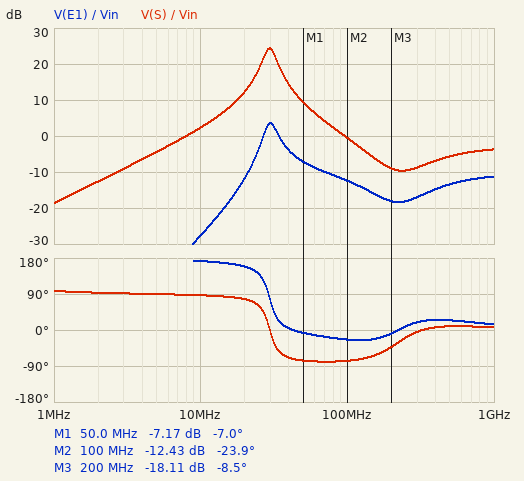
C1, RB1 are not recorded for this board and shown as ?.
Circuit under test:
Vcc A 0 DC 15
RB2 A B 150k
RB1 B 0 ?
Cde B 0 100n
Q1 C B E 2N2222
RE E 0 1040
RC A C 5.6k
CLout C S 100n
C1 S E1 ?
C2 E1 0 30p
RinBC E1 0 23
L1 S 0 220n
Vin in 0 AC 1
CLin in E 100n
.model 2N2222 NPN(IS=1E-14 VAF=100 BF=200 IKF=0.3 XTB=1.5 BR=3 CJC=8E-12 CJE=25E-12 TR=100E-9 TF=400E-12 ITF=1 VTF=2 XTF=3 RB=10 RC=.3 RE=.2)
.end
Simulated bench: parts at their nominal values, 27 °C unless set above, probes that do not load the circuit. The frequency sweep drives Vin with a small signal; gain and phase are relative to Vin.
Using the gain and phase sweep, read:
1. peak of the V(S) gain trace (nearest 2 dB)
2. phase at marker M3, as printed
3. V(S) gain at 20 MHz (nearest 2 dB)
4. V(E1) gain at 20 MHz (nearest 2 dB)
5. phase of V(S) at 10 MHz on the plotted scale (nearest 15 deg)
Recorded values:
24 dB
-8.5 deg
12 dB
-12 dB
90 deg
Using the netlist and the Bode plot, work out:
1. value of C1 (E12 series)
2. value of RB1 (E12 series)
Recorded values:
22 pF
47 kΩ
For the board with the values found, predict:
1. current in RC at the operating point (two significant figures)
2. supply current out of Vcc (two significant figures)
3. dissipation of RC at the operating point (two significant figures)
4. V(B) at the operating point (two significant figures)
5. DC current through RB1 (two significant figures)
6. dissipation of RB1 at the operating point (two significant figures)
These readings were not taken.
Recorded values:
2.2 mA
2.3 mA
28 mW
3.0 V
64 µA
190 µW
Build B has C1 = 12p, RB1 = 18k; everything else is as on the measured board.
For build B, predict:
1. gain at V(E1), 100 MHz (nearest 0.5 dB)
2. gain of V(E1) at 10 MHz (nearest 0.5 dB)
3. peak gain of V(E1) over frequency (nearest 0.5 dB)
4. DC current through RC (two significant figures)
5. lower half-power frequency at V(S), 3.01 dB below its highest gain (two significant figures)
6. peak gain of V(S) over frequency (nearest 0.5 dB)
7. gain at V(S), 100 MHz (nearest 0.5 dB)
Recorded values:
4.0 dB
-42.0 dB
11.0 dB
860 µA
79 MHz
28.5 dB
20.5 dB
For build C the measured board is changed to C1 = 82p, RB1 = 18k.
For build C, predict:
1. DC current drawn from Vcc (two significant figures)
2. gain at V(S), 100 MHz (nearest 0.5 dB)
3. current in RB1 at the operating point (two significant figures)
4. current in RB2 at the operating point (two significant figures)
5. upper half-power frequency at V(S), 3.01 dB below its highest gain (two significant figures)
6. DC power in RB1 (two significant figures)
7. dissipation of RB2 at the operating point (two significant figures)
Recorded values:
950 µA
1.0 dB
86 µA
90 µA
48 MHz
130 µW
1.2 mW
